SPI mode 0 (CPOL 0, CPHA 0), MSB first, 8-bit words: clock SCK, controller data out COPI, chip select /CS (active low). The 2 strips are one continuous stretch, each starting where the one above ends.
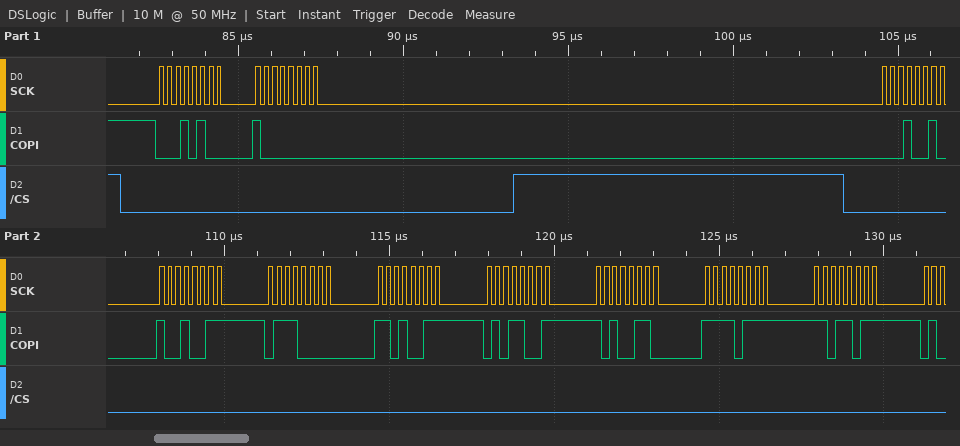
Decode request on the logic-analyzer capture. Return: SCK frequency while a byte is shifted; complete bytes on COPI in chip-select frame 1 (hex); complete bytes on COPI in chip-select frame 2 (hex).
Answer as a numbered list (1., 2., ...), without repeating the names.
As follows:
1. 4 MHz
2. 14 80
3. 12 93 70 D3 59 A6 F7 DB
